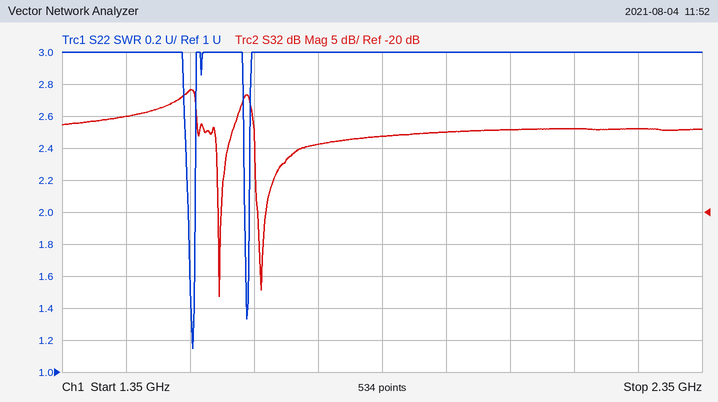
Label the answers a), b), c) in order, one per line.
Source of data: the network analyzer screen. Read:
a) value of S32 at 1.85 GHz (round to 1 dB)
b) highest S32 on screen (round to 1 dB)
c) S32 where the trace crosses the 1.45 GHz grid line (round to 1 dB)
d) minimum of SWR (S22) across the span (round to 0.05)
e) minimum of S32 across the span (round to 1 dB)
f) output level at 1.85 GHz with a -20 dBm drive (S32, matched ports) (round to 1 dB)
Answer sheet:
a) -8 dB
b) -1 dB
c) -5 dB
d) 1.15
e) -33 dB
f) -28 dBm
